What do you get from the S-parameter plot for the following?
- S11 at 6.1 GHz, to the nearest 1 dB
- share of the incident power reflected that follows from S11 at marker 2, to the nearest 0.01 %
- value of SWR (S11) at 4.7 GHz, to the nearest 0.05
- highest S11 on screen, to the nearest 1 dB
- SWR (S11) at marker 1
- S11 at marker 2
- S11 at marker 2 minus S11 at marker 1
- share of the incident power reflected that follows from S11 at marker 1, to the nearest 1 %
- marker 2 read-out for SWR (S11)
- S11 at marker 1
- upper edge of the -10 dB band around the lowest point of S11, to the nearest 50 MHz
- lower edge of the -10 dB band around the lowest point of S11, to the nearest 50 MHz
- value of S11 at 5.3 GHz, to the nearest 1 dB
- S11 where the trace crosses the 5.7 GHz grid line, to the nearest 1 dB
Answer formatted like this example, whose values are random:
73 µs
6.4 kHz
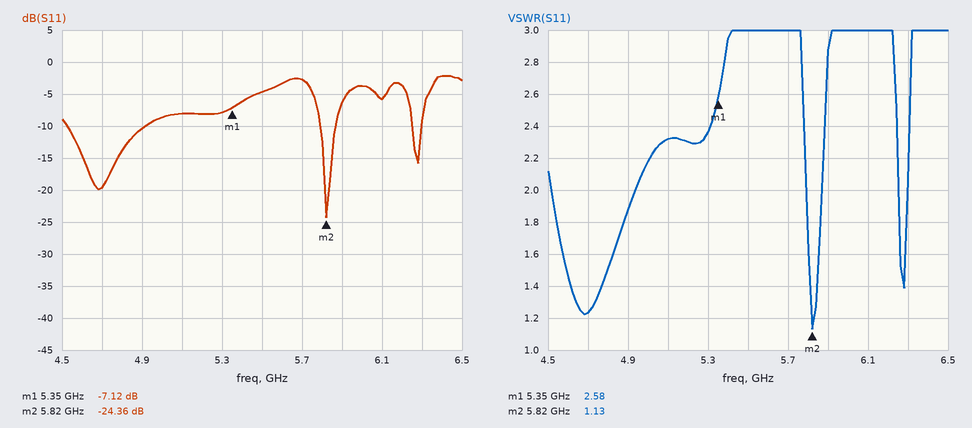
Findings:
-6 dB
0.37 %
1.25
-2 dB
2.58
-24.36 dB
-17.24 dB
19 %
1.13
-7.12 dB
5.85 GHz
5.80 GHz
-8 dB
-3 dB
